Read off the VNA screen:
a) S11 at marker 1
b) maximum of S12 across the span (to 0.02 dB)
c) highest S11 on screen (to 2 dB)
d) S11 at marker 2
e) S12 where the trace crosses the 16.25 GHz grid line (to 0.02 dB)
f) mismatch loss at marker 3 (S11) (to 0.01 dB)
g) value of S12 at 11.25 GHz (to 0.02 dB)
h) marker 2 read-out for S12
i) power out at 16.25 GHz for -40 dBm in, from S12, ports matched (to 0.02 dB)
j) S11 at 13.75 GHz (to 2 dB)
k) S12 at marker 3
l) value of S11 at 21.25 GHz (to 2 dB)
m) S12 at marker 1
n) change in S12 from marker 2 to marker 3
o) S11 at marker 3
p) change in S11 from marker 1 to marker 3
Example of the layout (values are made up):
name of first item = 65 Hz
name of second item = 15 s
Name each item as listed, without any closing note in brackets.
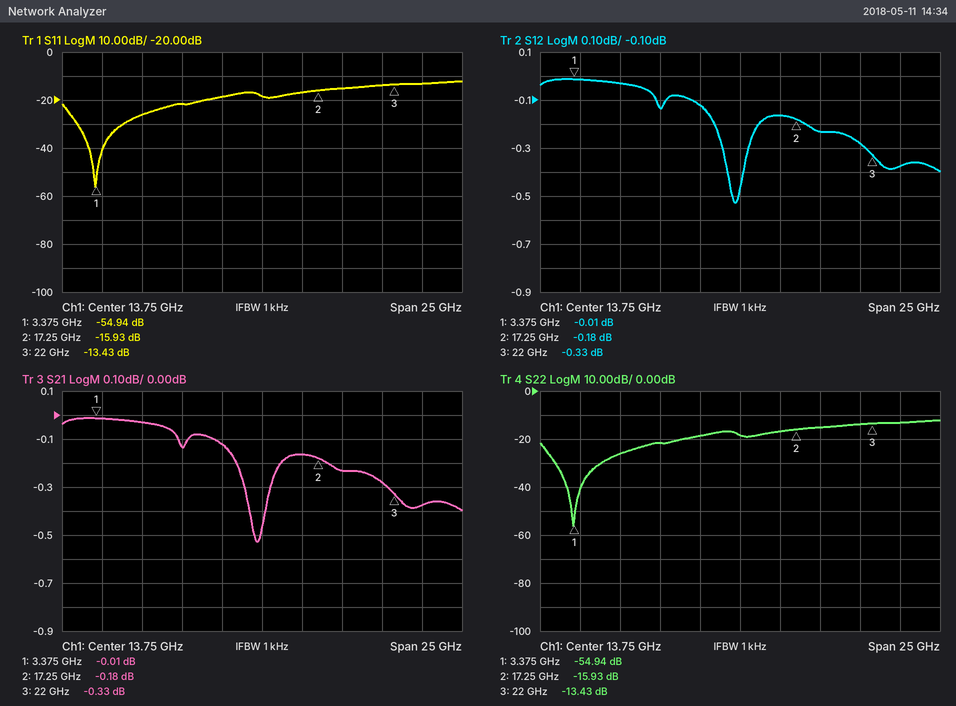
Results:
S11 at marker 1 = -54.94 dB
maximum of S12 across the span = -0.02 dB
highest S11 on screen = -12 dB
S11 at marker 2 = -15.93 dB
S12 where the trace crosses the 16.25 GHz grid line = -0.16 dB
mismatch loss at marker 3 (S11) = 0.20 dB
value of S12 at 11.25 GHz = -0.12 dB
marker 2 read-out for S12 = -0.18 dB
power out at 16.25 GHz for -40 dBm in, from S12, ports matched = -40.16 dBm
S11 at 13.75 GHz = -18 dB
S12 at marker 3 = -0.33 dB
value of S11 at 21.25 GHz = -14 dB
S12 at marker 1 = -0.01 dB
change in S12 from marker 2 to marker 3 = -0.15 dB
S11 at marker 3 = -13.43 dB
change in S11 from marker 1 to marker 3 = 41.51 dB
